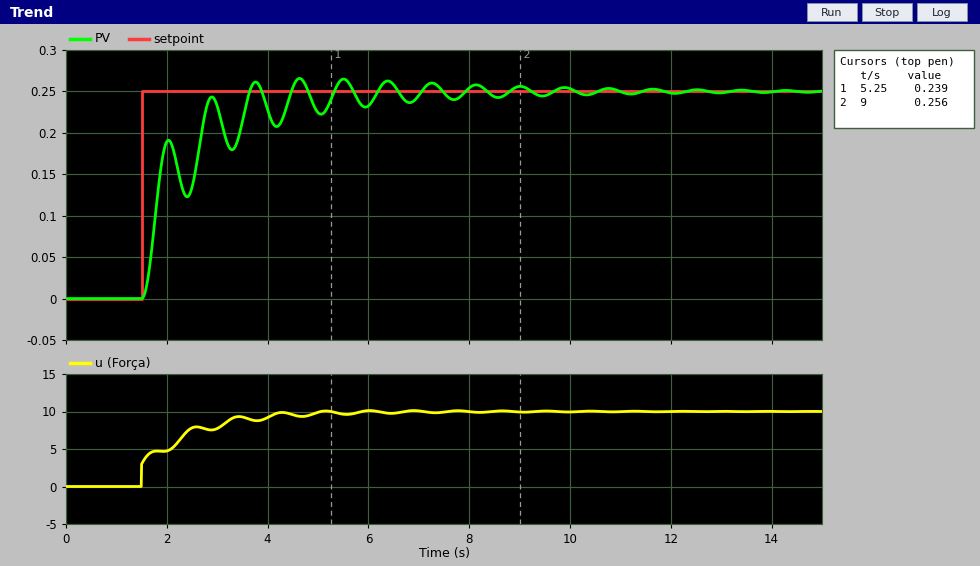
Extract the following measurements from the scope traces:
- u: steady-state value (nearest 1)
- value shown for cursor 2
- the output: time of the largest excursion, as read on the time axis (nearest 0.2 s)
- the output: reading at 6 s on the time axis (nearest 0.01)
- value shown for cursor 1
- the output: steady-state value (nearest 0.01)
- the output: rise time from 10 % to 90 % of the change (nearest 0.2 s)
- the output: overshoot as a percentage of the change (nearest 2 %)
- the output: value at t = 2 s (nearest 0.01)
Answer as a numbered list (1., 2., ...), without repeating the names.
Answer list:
1. 10
2. 0.256
3. 4.6 s
4. 0.23
5. 0.239
6. 0.25
7. 1.2 s
8. 6 %
9. 0.19
